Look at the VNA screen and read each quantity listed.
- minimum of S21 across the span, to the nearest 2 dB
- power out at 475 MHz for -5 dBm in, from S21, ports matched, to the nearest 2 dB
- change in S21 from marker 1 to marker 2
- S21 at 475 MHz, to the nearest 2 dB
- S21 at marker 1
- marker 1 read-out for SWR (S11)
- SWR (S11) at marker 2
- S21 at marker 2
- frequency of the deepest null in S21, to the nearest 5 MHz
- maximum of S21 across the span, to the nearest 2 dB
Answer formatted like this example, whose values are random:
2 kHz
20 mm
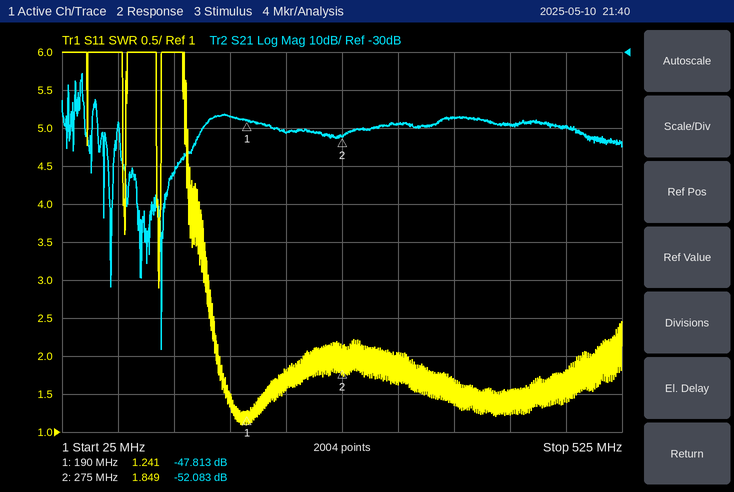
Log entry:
-108 dB
-54 dBm
-4.270 dB
-50 dB
-47.813 dB
1.241
1.849
-52.083 dB
115 MHz
-36 dB
